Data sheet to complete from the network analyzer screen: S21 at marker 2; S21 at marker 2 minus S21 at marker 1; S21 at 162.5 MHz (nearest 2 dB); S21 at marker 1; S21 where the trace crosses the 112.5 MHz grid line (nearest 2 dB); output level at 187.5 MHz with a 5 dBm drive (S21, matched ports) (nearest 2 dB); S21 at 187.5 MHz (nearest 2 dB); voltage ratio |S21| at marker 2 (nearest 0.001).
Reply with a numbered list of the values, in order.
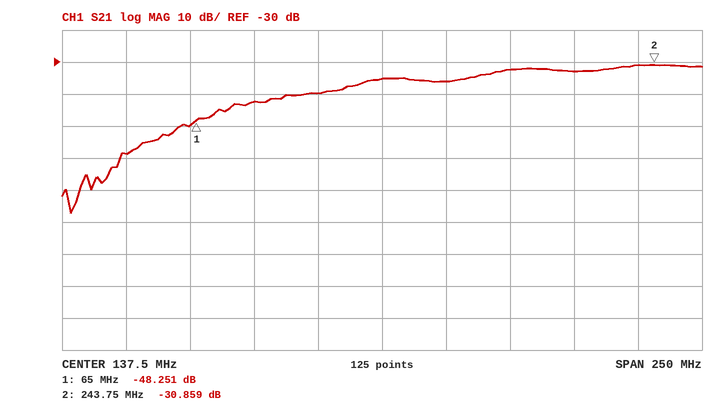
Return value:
1. -30.859 dB
2. 17.392 dB
3. -36 dB
4. -48.251 dB
5. -40 dB
6. -28 dBm
7. -32 dB
8. 0.029
